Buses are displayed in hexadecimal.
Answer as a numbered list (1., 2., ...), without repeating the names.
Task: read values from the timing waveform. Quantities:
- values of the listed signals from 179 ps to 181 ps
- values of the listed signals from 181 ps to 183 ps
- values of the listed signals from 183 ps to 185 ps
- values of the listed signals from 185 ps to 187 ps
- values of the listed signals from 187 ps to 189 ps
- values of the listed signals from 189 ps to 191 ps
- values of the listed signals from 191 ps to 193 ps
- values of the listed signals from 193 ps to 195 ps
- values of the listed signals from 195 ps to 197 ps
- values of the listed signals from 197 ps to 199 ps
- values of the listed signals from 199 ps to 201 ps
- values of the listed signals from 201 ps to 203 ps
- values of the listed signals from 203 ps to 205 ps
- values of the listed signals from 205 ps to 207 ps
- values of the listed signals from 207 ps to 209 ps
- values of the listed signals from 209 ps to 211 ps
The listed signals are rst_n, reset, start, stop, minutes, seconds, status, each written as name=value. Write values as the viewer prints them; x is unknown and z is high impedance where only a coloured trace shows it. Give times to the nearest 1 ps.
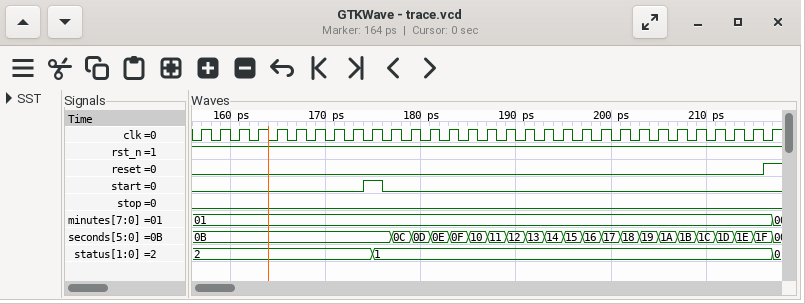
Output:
1. rst_n=1, reset=0, start=0, stop=0, minutes=01, seconds=0D, status=1
2. rst_n=1, reset=0, start=0, stop=0, minutes=01, seconds=0E, status=1
3. rst_n=1, reset=0, start=0, stop=0, minutes=01, seconds=0F, status=1
4. rst_n=1, reset=0, start=0, stop=0, minutes=01, seconds=10, status=1
5. rst_n=1, reset=0, start=0, stop=0, minutes=01, seconds=11, status=1
6. rst_n=1, reset=0, start=0, stop=0, minutes=01, seconds=12, status=1
7. rst_n=1, reset=0, start=0, stop=0, minutes=01, seconds=13, status=1
8. rst_n=1, reset=0, start=0, stop=0, minutes=01, seconds=14, status=1
9. rst_n=1, reset=0, start=0, stop=0, minutes=01, seconds=15, status=1
10. rst_n=1, reset=0, start=0, stop=0, minutes=01, seconds=16, status=1
11. rst_n=1, reset=0, start=0, stop=0, minutes=01, seconds=17, status=1
12. rst_n=1, reset=0, start=0, stop=0, minutes=01, seconds=18, status=1
13. rst_n=1, reset=0, start=0, stop=0, minutes=01, seconds=19, status=1
14. rst_n=1, reset=0, start=0, stop=0, minutes=01, seconds=1A, status=1
15. rst_n=1, reset=0, start=0, stop=0, minutes=01, seconds=1B, status=1
16. rst_n=1, reset=0, start=0, stop=0, minutes=01, seconds=1C, status=1
